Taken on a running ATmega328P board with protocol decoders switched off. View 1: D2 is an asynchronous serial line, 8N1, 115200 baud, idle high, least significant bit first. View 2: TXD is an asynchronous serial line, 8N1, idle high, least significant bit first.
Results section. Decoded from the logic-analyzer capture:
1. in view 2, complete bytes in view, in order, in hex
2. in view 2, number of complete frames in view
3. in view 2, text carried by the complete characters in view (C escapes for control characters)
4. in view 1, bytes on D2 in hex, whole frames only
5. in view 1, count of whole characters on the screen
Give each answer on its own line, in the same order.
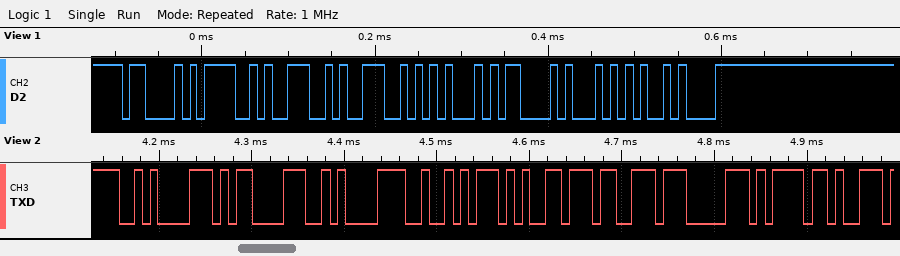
0A 0D 0A 52 65 73 70 6F
8
"\n\r\nRespo"
0x43 0x4F 0x4E 0x4E 0x45 0x43 0x54 0x0A
8
